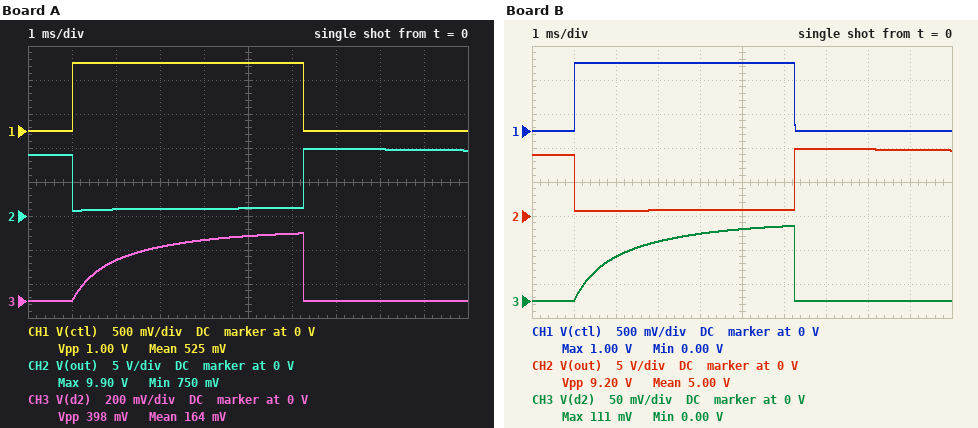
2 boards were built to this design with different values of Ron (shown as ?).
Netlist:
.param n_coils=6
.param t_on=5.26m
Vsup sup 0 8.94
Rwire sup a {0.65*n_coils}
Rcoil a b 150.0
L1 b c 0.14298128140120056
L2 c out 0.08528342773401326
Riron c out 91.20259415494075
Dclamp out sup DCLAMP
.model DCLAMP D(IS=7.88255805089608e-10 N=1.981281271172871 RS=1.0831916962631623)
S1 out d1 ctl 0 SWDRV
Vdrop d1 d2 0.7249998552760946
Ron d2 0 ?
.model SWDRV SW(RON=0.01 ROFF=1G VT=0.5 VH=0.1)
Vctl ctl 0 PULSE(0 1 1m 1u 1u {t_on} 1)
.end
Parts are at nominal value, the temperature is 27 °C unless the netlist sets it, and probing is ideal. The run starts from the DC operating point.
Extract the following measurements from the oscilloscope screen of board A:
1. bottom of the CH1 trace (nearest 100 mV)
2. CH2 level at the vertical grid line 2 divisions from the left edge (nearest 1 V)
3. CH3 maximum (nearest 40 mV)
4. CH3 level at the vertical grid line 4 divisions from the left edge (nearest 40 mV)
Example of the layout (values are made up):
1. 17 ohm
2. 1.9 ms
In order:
1. 0 V
2. 1 V
3. 400 mV
4. 360 mV
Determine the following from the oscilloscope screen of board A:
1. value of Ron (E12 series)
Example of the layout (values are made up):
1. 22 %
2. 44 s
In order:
1. 8.2 Ω
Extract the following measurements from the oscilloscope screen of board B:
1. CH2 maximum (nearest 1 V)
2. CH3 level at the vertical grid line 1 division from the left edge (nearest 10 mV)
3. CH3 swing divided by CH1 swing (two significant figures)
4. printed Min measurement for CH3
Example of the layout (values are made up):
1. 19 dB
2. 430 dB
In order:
1. 10 V
2. 0 V
3. 0.11
4. 0.00 V
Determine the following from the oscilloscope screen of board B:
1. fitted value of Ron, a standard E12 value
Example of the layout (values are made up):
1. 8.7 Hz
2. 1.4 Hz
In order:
1. 2.2 Ω
